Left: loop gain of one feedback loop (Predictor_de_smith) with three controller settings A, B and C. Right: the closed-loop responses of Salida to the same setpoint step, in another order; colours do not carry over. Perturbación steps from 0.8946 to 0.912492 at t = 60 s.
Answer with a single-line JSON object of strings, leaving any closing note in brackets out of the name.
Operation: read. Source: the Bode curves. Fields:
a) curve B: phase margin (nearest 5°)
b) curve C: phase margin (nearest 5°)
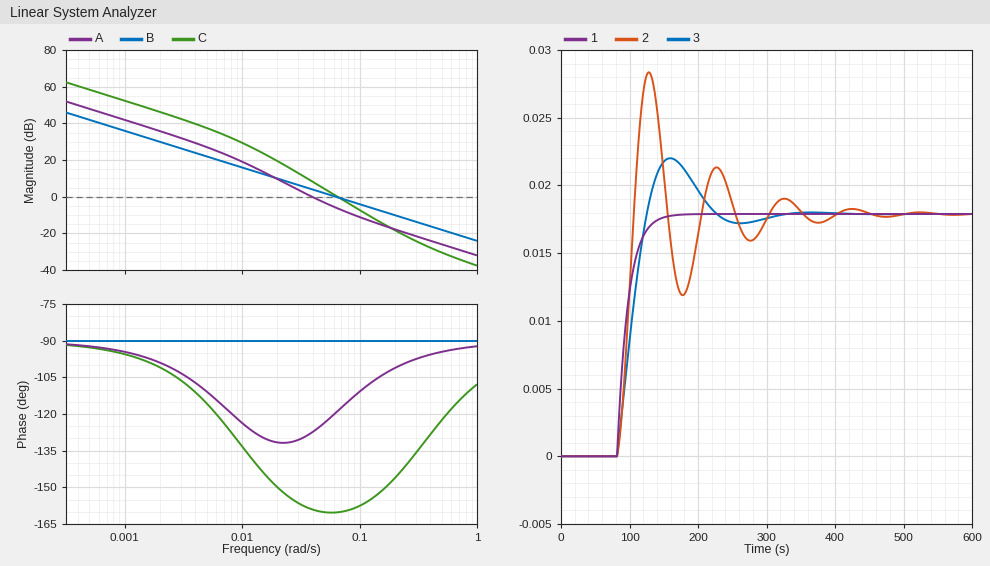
{"curve B: phase margin": "90°", "curve C: phase margin": "20°"}
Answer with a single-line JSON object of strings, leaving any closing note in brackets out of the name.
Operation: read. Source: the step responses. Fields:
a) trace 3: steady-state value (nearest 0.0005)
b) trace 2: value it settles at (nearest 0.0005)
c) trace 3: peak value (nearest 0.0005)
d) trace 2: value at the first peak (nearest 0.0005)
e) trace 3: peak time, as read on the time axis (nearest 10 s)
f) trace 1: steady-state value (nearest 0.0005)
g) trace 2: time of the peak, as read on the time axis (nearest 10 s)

{"trace 3: steady-state value": "0.0180", "trace 2: value it settles at": "0.0180", "trace 3: peak value": "0.0220", "trace 2: value at the first peak": "0.0285", "trace 3: peak time, as read on the time axis": "160 s", "trace 1: steady-state value": "0.0180", "trace 2: time of the peak, as read on the time axis": "130 s"}
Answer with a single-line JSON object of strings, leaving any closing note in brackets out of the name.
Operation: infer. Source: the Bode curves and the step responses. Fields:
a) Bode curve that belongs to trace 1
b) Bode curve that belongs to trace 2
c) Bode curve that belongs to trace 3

{"Bode curve that belongs to trace 1": "B", "Bode curve that belongs to trace 2": "C", "Bode curve that belongs to trace 3": "A"}
